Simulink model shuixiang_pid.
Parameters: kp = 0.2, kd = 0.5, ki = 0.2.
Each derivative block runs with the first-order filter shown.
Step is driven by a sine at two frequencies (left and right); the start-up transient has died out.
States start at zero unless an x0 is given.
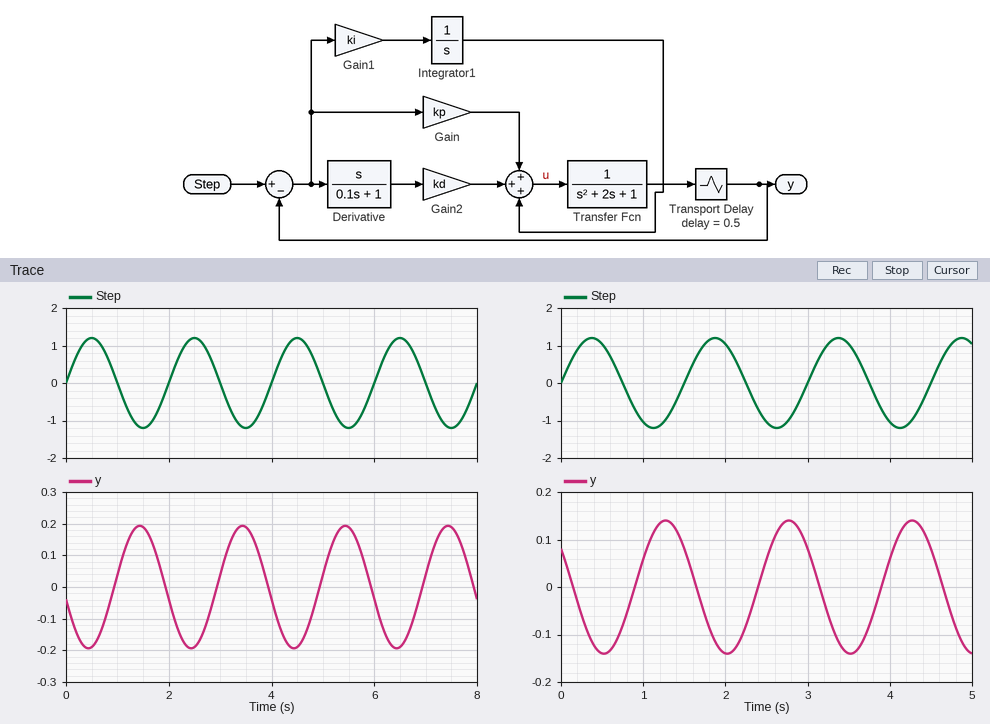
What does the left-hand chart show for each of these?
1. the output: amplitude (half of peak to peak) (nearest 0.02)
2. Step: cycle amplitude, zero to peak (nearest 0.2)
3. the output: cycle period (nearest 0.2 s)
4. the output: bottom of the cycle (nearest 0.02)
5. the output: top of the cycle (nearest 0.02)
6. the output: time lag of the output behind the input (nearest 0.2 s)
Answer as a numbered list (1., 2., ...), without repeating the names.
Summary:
1. 0.20
2. 1.2
3. 2.0 s
4. -0.20
5. 0.20
6. 1.0 s
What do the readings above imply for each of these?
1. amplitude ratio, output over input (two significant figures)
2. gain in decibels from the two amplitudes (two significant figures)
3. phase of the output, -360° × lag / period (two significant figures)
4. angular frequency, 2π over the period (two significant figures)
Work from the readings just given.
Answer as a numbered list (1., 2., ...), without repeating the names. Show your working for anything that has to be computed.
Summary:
1. 0.2 / 1.2 = 0.17
2. 20 log10(0.2 / 1.2) = -16 dB
3. -360 × 1 / 2 = -180°
4. 2π / 2 = 3.1 rad/s
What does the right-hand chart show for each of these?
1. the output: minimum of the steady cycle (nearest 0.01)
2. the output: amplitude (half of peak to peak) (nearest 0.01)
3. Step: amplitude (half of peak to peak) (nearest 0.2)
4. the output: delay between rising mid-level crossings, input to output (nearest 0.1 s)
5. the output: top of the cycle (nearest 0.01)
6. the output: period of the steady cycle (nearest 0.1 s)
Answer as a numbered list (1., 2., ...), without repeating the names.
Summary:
1. -0.14
2. 0.14
3. 1.2
4. 0.9 s
5. 0.14
6. 1.5 s
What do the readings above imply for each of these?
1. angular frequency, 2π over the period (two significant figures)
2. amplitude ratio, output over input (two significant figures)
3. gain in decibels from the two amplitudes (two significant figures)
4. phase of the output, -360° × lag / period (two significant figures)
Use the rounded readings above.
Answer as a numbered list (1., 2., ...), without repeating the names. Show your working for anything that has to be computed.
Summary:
1. 2π / 1.5 = 4.2 rad/s
2. 0.14 / 1.2 = 0.12
3. 20 log10(0.14 / 1.2) = -19 dB
4. -360 × 0.9 / 1.5 = -220°
